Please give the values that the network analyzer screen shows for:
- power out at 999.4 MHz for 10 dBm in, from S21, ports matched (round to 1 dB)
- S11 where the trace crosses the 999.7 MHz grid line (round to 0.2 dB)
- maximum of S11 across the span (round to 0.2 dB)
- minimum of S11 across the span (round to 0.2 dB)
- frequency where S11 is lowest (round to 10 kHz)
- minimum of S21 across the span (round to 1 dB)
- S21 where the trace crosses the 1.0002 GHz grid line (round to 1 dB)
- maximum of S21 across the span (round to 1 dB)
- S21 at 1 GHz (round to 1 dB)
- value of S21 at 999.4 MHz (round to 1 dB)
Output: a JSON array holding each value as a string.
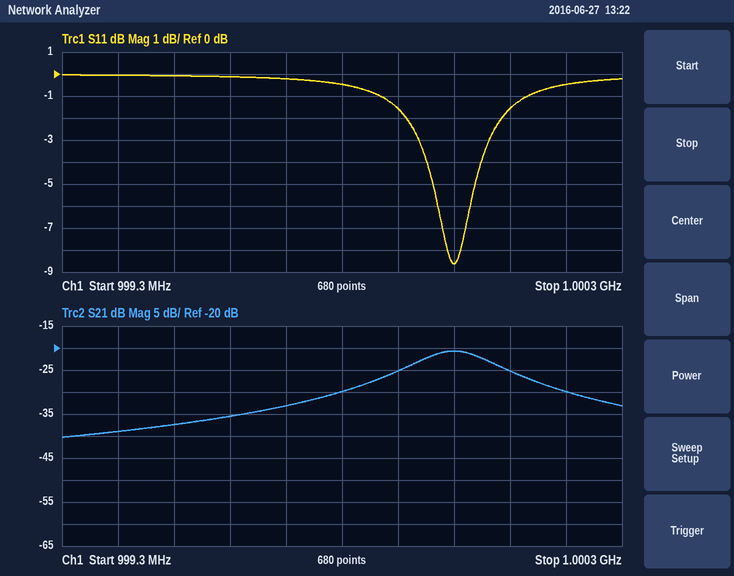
["-29 dBm", "-0.2 dB", "0.0 dB", "-8.6 dB", "1.00000 GHz", "-40 dB", "-30 dB", "-21 dB", "-21 dB", "-39 dB"]
